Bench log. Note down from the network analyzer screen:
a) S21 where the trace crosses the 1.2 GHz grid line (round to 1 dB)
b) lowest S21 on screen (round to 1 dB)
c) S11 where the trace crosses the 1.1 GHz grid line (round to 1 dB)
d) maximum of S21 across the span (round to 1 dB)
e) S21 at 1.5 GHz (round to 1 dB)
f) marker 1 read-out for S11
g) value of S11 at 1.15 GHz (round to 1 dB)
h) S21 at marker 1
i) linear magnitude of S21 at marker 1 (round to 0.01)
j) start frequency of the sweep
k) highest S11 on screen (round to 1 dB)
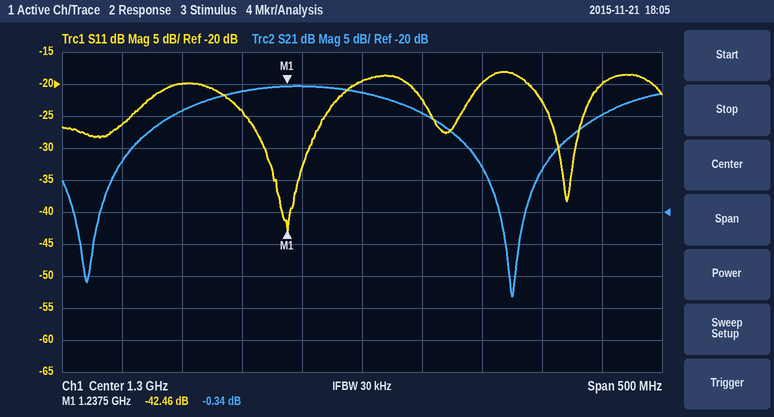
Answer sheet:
-1 dB
-33 dB
-26 dB
0 dB
-5 dB
-42.46 dB
-20 dB
-0.34 dB
0.96
1.05 GHz
-18 dB
